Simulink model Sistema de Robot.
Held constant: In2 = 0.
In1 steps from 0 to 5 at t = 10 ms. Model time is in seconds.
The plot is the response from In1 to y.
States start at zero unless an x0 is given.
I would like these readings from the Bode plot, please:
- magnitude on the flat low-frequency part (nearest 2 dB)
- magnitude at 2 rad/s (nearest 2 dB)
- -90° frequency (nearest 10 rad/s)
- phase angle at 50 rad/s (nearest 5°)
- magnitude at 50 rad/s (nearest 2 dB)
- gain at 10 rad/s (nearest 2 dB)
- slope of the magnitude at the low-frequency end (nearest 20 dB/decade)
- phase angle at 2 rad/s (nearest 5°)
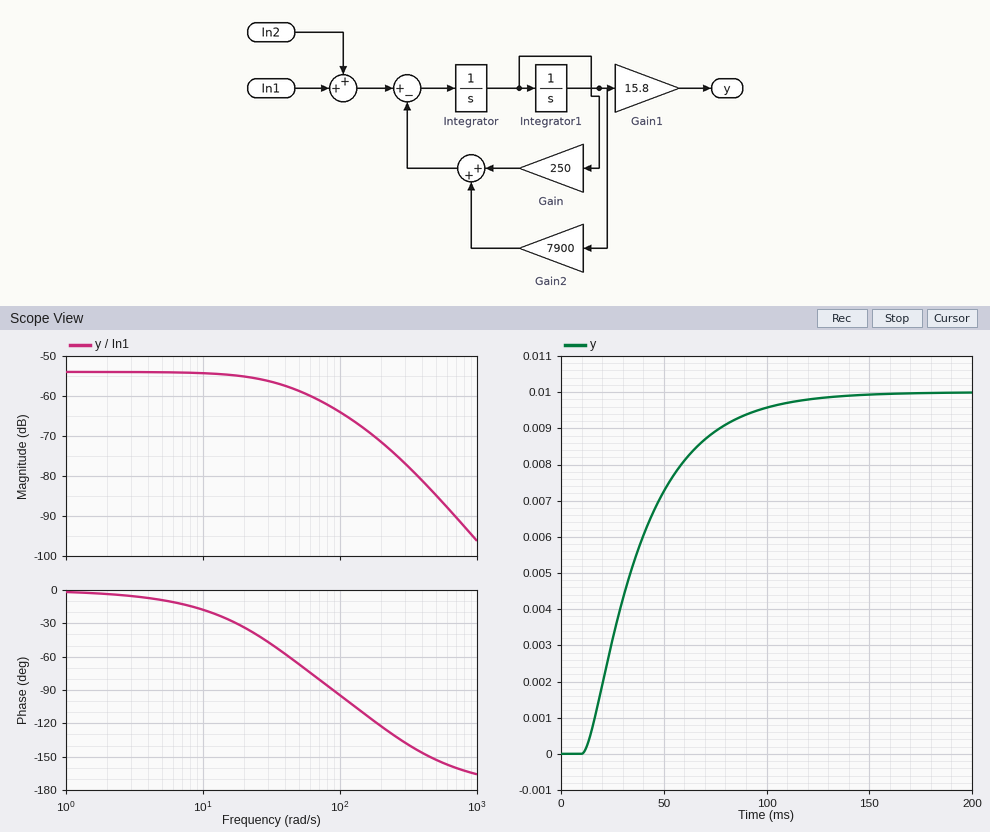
-54 dB
-54 dB
90 rad/s
-65°
-58 dB
-54 dB
0 dB/decade
-5°
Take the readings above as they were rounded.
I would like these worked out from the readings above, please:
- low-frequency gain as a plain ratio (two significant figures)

0.0020
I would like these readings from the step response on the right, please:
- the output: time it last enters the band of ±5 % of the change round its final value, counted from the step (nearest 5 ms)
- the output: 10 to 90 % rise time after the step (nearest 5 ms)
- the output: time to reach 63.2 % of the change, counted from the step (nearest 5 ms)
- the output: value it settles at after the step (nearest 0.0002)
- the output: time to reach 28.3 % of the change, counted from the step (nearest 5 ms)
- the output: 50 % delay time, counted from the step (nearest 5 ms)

85 ms
60 ms
30 ms
0.0100
15 ms
25 ms
